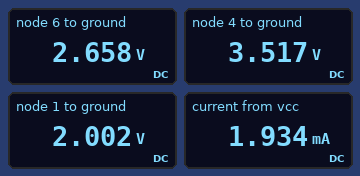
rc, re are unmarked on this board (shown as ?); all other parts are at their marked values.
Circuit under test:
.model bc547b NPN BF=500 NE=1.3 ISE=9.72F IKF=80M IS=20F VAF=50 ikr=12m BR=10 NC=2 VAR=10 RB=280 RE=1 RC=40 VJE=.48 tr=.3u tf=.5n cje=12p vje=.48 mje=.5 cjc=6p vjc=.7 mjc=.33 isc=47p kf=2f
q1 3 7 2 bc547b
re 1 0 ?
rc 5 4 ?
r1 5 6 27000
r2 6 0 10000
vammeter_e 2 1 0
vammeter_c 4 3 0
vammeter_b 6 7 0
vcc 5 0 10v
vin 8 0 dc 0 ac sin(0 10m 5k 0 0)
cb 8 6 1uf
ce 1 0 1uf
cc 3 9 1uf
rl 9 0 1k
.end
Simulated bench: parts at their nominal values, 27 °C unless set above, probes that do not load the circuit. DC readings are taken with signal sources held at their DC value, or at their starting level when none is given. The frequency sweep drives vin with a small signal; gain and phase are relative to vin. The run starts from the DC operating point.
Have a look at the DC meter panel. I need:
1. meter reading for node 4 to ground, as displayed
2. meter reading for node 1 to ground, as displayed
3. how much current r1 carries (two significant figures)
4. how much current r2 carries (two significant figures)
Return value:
3.517 V
2.002 V
270 µA
270 µA
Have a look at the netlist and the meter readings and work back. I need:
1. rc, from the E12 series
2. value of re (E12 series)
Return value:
3.9 kΩ
1.2 kΩ
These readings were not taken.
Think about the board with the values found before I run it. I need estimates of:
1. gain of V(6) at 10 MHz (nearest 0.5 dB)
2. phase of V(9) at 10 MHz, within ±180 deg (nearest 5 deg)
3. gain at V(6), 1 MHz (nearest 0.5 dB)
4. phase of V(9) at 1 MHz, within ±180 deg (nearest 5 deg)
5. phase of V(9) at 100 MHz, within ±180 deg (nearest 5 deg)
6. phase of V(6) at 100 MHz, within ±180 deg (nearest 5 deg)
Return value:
0 dB
100 deg
0 dB
155 deg
65 deg
0 deg
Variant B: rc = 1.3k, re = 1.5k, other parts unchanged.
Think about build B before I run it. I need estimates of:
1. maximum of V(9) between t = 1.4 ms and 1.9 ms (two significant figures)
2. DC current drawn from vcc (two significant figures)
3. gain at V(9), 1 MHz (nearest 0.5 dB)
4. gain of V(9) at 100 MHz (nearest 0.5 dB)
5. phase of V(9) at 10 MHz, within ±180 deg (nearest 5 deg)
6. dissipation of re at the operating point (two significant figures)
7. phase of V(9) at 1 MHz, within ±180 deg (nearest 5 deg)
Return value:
140 mV
1.6 mA
28.0 dB
0 dB
110 deg
2.7 mW
165 deg
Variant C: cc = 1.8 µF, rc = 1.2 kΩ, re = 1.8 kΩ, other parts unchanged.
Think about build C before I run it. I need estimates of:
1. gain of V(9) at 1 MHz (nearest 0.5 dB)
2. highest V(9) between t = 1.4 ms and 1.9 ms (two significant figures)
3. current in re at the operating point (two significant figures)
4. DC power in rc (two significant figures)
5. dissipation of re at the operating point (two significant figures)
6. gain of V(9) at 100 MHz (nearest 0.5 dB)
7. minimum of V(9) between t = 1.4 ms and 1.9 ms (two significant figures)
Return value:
26.5 dB
130 mV
1.1 mA
1.5 mW
2.3 mW
-0.5 dB
-140 mV
